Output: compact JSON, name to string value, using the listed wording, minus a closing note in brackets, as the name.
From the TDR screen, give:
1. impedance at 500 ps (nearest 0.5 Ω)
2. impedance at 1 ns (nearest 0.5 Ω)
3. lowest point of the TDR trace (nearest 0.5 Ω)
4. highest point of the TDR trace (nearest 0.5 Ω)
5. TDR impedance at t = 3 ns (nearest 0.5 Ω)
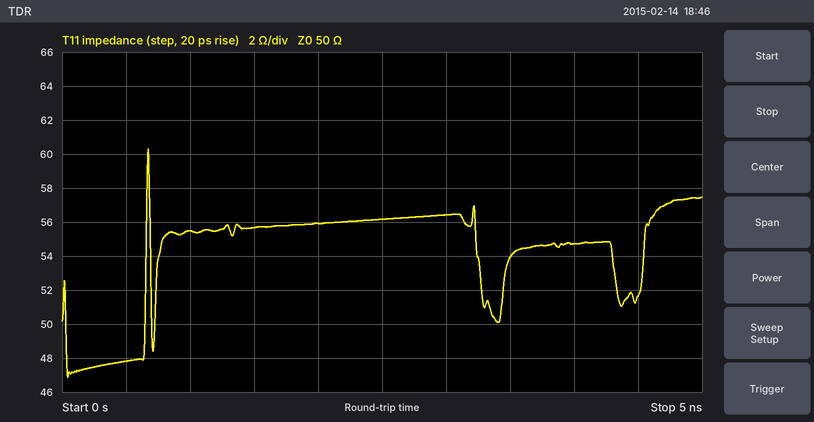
{"impedance at 500 ps": "48.0 Ω", "impedance at 1 ns": "55.5 Ω", "lowest point of the TDR trace": "47.0 Ω", "highest point of the TDR trace": "60.5 Ω", "TDR impedance at t = 3 ns": "56.5 Ω"}
